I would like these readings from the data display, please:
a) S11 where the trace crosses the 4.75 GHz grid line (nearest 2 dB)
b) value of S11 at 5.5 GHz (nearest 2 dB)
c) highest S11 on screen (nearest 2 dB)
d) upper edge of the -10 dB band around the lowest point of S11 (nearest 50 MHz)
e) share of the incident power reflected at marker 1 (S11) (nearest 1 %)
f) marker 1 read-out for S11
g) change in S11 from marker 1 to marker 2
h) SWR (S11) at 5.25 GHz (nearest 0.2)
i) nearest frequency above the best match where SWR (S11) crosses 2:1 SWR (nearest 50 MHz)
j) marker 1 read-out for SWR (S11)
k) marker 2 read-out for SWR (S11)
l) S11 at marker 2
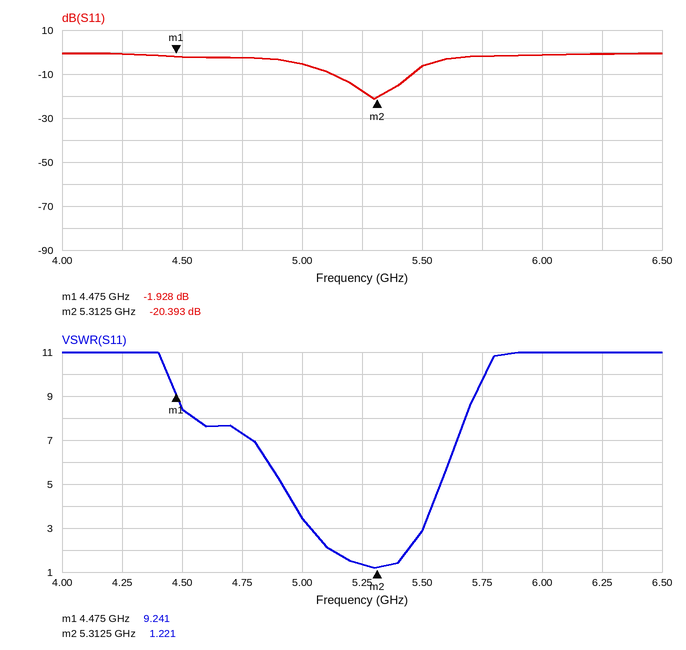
-2 dB
-6 dB
0 dB
5.45 GHz
64 %
-1.928 dB
-18.465 dB
1.4
5.45 GHz
9.241
1.221
-20.393 dB
